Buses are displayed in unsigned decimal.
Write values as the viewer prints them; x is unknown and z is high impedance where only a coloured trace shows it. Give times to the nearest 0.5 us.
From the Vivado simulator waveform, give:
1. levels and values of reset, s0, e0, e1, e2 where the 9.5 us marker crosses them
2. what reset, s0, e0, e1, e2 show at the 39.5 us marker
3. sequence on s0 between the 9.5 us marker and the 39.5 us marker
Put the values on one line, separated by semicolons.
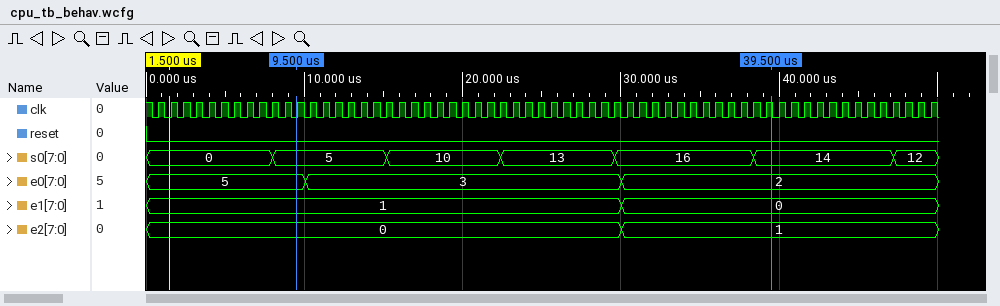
reset=0, s0=5, e0=5, e1=1, e2=0; reset=0, s0=14, e0=2, e1=0, e2=1; 5, 10, 13, 16, 14
